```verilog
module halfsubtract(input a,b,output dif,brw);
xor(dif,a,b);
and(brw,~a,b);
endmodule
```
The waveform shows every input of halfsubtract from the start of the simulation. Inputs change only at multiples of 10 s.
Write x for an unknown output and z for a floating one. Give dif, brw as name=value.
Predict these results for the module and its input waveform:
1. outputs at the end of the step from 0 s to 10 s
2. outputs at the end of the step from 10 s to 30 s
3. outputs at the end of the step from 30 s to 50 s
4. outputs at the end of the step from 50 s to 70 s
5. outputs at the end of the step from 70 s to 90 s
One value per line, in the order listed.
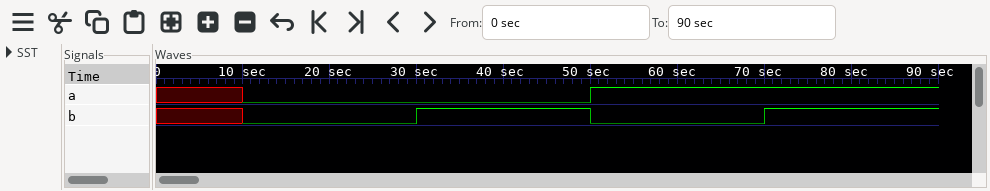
dif=x, brw=x
dif=0, brw=0
dif=1, brw=1
dif=1, brw=0
dif=0, brw=0
